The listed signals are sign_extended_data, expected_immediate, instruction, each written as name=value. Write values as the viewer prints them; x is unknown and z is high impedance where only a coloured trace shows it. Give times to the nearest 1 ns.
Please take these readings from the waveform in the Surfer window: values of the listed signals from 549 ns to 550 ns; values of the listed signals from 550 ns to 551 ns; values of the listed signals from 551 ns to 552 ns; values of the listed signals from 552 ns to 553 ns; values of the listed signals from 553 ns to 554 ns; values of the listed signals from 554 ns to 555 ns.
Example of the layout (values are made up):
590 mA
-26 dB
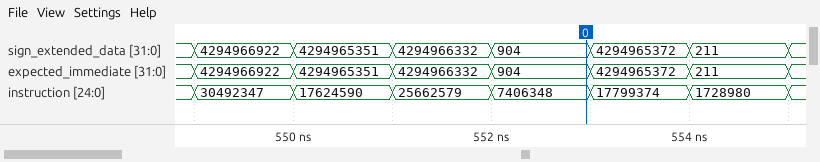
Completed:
sign_extended_data=4294966922, expected_immediate=4294966922, instruction=30492347
sign_extended_data=4294965351, expected_immediate=4294965351, instruction=17624590
sign_extended_data=4294966332, expected_immediate=4294966332, instruction=25662579
sign_extended_data=904, expected_immediate=904, instruction=7406348
sign_extended_data=4294965372, expected_immediate=4294965372, instruction=17799374
sign_extended_data=211, expected_immediate=211, instruction=1728980
